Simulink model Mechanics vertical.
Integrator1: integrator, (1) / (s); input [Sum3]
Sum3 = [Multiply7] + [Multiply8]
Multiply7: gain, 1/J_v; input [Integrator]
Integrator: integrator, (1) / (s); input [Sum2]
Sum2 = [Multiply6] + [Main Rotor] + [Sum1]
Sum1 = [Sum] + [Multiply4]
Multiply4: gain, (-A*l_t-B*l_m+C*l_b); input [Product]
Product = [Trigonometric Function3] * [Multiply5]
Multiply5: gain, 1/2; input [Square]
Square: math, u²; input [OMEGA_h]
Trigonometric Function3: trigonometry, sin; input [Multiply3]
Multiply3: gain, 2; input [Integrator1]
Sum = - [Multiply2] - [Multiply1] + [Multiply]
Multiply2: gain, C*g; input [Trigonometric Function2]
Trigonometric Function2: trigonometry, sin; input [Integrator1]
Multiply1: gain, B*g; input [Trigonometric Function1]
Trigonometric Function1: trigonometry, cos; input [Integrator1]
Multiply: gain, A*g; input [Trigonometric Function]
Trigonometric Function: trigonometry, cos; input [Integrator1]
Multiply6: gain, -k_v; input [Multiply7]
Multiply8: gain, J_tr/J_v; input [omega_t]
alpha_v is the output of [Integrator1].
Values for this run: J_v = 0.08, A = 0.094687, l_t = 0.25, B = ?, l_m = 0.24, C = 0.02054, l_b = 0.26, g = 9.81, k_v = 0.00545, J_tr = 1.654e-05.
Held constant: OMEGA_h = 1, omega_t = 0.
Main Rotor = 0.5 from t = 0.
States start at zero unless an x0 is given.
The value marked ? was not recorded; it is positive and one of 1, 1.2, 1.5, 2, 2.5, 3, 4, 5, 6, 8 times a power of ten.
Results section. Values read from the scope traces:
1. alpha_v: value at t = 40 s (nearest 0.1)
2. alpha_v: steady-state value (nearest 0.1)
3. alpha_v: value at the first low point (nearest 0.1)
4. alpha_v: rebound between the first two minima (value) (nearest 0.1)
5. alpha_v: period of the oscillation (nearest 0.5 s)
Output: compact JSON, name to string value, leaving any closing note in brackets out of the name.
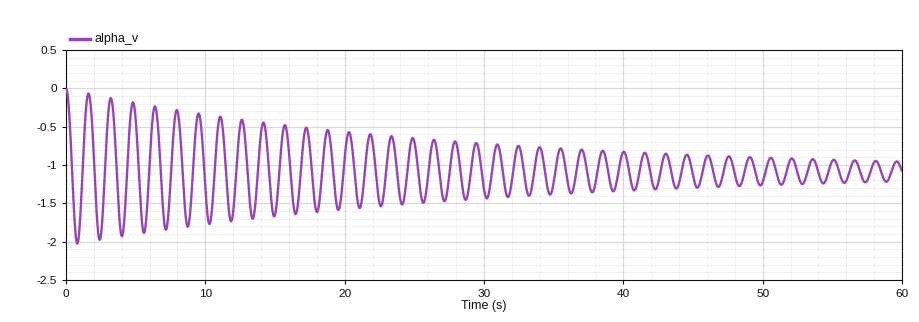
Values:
{"alpha_v: value at t = 40 s": "-0.8", "alpha_v: steady-state value": "-1.1", "alpha_v: value at the first low point": "-2.0", "alpha_v: rebound between the first two minima (value)": "-0.1", "alpha_v: period of the oscillation": "1.5 s"}
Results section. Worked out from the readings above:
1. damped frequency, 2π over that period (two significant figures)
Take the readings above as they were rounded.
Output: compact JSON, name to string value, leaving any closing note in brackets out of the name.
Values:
{"damped frequency, 2π over that period": "4.2 rad/s"}
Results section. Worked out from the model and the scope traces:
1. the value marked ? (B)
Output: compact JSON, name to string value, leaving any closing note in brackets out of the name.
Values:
{"the value marked ?": "0.25"}
